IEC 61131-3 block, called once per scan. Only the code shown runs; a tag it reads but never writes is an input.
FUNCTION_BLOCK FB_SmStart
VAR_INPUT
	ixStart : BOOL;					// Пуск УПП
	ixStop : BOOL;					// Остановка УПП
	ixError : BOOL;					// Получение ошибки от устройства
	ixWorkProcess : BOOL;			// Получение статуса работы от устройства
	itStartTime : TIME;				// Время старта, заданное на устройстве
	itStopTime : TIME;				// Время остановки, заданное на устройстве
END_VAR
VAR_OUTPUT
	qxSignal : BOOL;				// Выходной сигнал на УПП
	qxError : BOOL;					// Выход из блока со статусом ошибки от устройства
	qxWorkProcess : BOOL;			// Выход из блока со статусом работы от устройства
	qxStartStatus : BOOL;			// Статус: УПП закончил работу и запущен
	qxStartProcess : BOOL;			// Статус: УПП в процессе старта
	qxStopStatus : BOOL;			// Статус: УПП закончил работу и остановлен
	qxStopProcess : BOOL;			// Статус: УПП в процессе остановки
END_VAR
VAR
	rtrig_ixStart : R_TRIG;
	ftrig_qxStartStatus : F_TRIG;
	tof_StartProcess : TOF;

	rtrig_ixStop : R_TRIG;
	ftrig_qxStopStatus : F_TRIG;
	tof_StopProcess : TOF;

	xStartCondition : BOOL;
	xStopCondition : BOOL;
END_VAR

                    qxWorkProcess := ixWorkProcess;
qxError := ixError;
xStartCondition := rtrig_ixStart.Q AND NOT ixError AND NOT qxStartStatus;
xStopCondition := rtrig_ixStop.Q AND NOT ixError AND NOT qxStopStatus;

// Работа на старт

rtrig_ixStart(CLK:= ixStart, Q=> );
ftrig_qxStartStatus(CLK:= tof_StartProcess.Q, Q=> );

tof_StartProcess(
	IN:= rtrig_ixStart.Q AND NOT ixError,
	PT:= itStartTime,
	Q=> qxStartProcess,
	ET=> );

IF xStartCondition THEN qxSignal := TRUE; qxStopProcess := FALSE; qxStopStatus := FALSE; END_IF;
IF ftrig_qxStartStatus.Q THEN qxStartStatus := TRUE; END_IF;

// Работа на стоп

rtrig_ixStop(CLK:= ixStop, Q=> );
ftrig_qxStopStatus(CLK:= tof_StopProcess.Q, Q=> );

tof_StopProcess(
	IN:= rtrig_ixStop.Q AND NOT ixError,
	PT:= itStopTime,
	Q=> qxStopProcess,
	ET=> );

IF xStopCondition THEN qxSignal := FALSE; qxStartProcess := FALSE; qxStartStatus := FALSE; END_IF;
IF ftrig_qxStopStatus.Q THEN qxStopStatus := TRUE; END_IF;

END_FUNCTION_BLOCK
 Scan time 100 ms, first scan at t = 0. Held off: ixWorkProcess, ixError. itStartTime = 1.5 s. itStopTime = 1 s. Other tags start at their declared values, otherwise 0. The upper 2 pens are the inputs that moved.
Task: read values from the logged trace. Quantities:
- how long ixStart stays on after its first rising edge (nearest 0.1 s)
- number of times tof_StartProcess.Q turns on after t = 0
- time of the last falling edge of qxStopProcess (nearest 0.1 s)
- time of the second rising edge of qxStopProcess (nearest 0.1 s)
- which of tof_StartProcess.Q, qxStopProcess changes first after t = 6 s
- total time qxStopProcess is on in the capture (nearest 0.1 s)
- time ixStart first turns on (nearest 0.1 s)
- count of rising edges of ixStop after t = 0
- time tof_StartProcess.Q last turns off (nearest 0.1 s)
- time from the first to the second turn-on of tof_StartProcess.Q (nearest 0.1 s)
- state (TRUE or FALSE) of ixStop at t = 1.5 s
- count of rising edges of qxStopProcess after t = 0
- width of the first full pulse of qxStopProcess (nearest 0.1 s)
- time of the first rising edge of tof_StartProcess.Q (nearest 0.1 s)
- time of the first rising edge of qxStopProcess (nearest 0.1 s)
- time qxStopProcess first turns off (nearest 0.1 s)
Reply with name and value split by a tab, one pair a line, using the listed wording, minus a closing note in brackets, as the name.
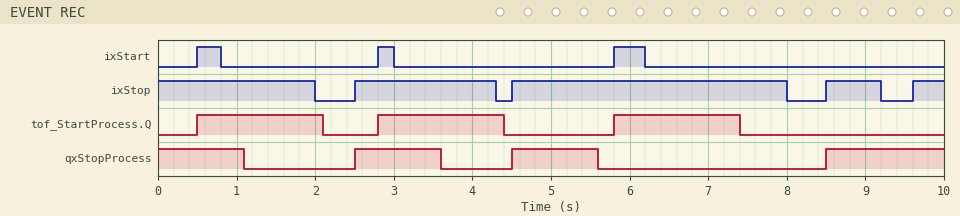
how long ixStart stays on after its first rising edge	0.3 s
number of times tof_StartProcess.Q turns on after t = 0	3
time of the last falling edge of qxStopProcess	5.6 s
time of the second rising edge of qxStopProcess	4.5 s
which of tof_StartProcess.Q, qxStopProcess changes first after t = 6 s	tof_StartProcess.Q
total time qxStopProcess is on in the capture	4.8 s
time ixStart first turns on	0.5 s
count of rising edges of ixStop after t = 0	4
time tof_StartProcess.Q last turns off	7.4 s
time from the first to the second turn-on of tof_StartProcess.Q	2.3 s
state (TRUE or FALSE) of ixStop at t = 1.5 s	TRUE
count of rising edges of qxStopProcess after t = 0	3
width of the first full pulse of qxStopProcess	1.1 s
time of the first rising edge of tof_StartProcess.Q	0.5 s
time of the first rising edge of qxStopProcess	2.5 s
time qxStopProcess first turns off	1.1 s
